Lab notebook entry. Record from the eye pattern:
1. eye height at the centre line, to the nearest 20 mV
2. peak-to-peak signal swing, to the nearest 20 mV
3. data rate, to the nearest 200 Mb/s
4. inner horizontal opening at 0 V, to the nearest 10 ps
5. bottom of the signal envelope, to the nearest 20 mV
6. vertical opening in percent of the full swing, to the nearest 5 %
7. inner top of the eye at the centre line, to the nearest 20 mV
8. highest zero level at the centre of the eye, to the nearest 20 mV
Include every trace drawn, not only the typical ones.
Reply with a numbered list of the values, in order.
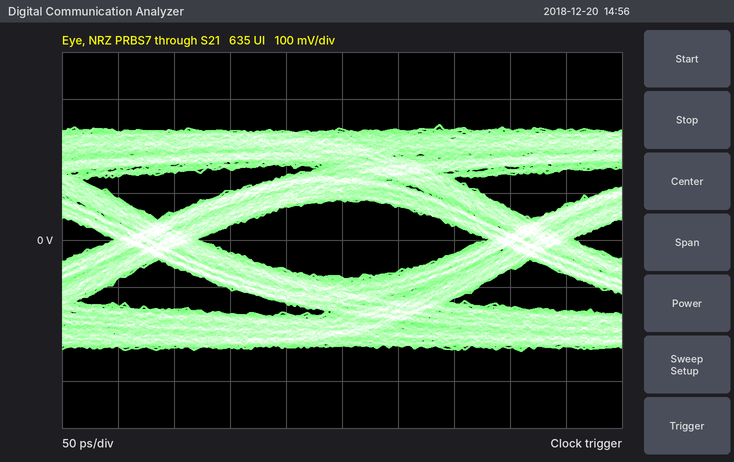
1. 160 mV
2. 480 mV
3. 3.0 Gb/s
4. 260 ps
5. -240 mV
6. 35 %
7. 80 mV
8. -80 mV
